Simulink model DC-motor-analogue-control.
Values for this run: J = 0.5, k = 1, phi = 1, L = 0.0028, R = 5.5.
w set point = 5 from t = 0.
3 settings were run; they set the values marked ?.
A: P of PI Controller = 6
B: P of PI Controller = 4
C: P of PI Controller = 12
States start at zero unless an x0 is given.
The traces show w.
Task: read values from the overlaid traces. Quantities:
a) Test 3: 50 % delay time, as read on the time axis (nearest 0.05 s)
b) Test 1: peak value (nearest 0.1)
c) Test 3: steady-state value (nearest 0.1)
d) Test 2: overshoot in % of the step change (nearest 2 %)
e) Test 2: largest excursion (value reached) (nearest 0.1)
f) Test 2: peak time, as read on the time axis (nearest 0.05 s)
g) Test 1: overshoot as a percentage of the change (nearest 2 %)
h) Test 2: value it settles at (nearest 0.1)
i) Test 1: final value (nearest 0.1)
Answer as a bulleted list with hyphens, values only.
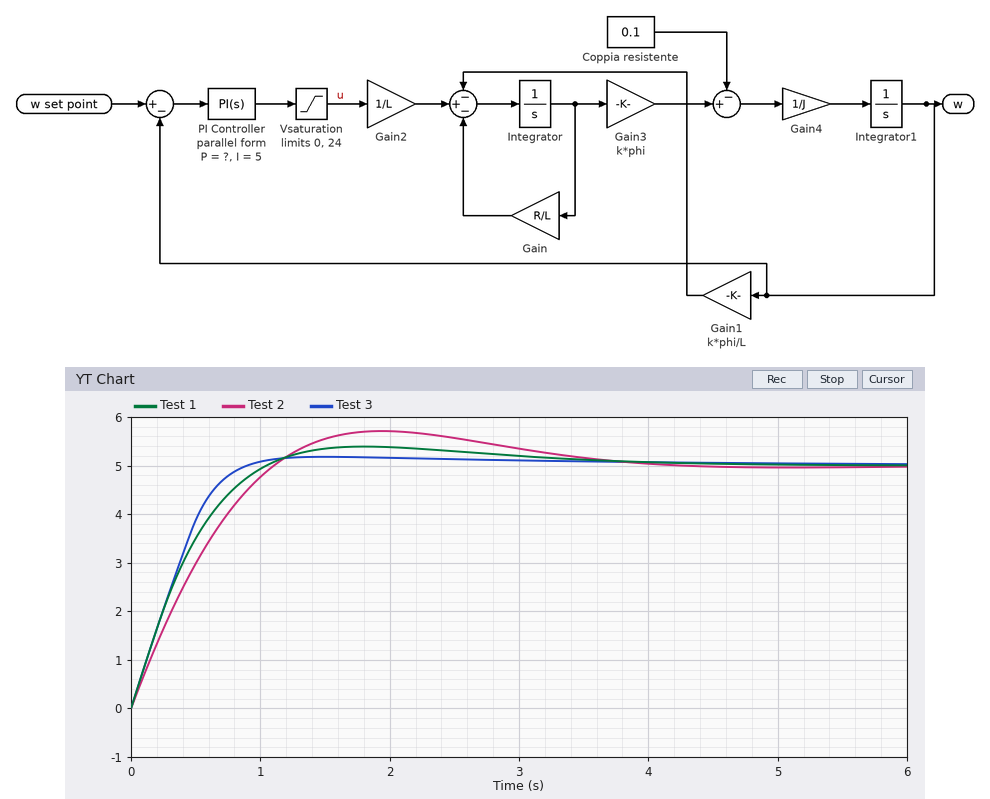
- 0.30 s
- 5.4
- 5.0
- 14 %
- 5.7
- 1.95 s
- 8 %
- 5.0
- 5.0
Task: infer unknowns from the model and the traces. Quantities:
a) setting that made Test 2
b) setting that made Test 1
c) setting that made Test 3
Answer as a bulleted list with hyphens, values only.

- B
- A
- C
